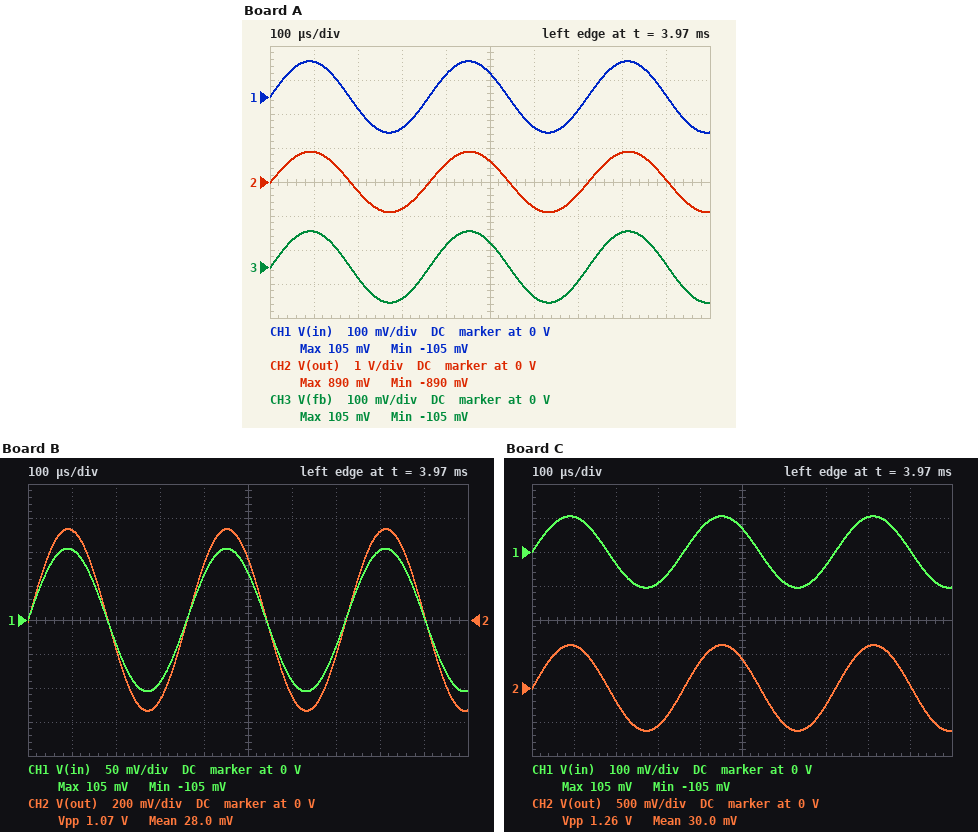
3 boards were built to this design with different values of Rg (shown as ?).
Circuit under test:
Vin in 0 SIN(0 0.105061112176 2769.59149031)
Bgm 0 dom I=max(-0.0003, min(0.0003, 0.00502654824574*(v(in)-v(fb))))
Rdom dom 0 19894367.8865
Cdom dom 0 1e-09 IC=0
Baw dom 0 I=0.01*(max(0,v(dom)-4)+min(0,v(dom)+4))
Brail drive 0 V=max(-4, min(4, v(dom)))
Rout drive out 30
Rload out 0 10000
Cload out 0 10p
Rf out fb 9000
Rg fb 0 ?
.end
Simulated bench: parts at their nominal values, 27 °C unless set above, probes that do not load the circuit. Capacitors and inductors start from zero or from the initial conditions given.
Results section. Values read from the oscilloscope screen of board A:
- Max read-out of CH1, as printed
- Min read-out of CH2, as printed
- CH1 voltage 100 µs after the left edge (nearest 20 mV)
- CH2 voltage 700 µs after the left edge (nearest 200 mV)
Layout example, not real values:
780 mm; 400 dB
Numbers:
105 mV; -890 mV; 100 mV; -400 mV
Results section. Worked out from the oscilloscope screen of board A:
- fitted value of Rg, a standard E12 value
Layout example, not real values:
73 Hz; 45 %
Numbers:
1.2 kΩ
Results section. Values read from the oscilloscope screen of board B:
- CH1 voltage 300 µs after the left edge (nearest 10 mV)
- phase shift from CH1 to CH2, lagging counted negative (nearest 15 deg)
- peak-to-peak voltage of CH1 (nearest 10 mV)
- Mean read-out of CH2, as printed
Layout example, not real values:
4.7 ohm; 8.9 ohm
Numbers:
-90 mV; 0 deg; 210 mV; 28.0 mV
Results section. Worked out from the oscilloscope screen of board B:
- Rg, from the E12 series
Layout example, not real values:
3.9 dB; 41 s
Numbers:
2.2 kΩ
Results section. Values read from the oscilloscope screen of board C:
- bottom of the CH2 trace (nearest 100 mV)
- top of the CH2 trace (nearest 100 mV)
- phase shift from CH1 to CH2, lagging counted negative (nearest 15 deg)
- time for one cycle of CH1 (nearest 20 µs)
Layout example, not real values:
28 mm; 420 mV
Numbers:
-600 mV; 600 mV; 0 deg; 360 µs
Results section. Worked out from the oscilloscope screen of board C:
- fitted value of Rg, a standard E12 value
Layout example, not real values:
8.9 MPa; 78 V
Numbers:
1.8 kΩ
